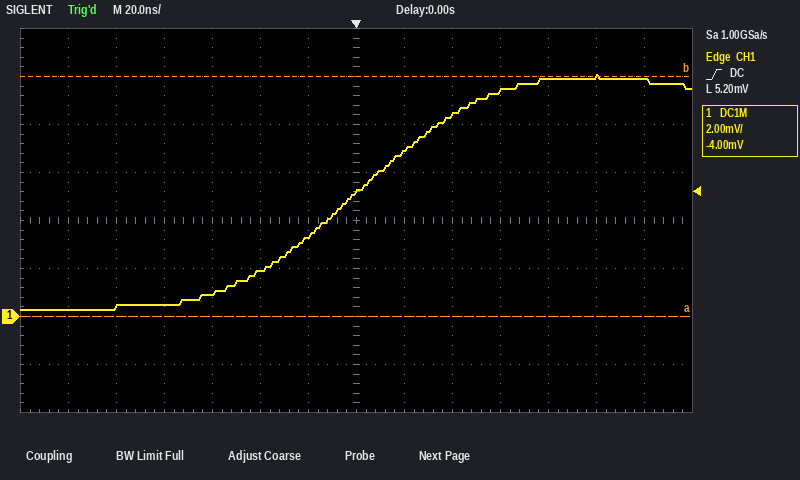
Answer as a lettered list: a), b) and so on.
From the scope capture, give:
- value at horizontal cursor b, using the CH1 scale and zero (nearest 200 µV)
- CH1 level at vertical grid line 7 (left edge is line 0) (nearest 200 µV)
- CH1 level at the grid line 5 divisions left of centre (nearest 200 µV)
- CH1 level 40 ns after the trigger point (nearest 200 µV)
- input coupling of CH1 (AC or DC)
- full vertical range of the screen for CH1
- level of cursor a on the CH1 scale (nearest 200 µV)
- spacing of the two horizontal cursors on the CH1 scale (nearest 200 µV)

a) 10.0 mV
b) 5.2 mV
c) 400 µV
d) 8.4 mV
e) DC
f) 16 mV
g) 0.0 mV
h) 10.0 mV
